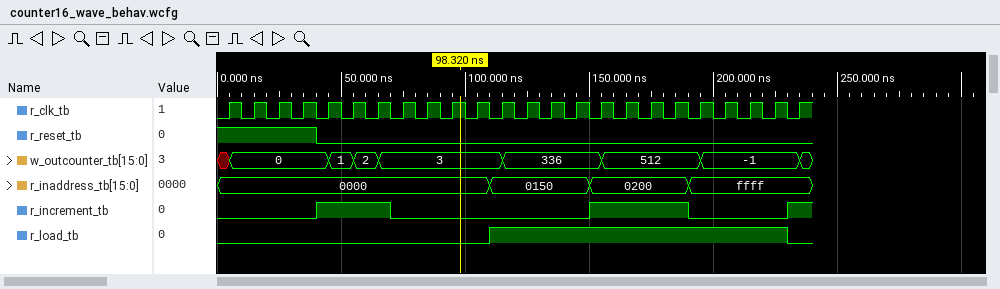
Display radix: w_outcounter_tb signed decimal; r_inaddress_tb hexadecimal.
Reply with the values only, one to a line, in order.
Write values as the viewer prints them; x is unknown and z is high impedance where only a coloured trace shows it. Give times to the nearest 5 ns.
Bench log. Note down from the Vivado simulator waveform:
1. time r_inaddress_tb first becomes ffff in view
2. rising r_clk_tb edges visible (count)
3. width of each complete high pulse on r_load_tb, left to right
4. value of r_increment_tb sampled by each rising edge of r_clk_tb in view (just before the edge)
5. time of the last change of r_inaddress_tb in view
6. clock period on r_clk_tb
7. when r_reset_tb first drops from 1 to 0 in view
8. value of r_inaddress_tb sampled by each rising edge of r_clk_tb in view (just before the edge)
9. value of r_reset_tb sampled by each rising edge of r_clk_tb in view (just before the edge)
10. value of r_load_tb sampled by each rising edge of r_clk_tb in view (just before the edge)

190 ns
24
120 ns
0 0 0 0 1 1 1 0 0 0 0 0 0 0 0 1 1 1 1 0 0 0 0 1
190 ns
10 ns
40 ns
0000, 0000, 0000, 0000, 0000, 0000, 0000, 0000, 0000, 0000, 0000, 0150, 0150, 0150, 0150, 0200, 0200, 0200, 0200, ffff, ffff, ffff, ffff, ffff
1 1 1 1 0 0 0 0 0 0 0 0 0 0 0 0 0 0 0 0 0 0 0 0
0 0 0 0 0 0 0 0 0 0 0 1 1 1 1 1 1 1 1 1 1 1 1 0
